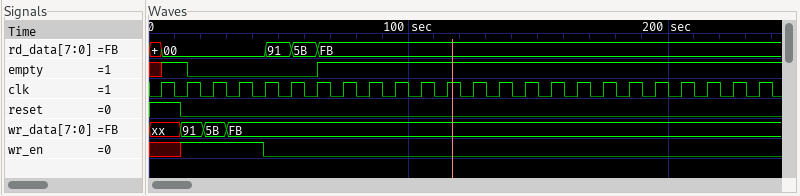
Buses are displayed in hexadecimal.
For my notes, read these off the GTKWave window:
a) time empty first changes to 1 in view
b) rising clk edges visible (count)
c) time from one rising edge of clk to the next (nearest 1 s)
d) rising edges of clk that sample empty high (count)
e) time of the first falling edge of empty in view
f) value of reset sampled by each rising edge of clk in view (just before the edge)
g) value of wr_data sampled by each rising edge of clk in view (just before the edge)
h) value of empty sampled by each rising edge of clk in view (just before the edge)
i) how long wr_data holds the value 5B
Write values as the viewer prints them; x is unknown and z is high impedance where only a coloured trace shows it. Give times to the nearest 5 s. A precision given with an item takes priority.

5 s
24
10 s
18
15 s
1 0 0 0 0 0 0 0 0 0 0 0 0 0 0 0 0 0 0 0 0 0 0 0
xx, 91, 5B, FB, FB, FB, FB, FB, FB, FB, FB, FB, FB, FB, FB, FB, FB, FB, FB, FB, FB, FB, FB, FB
x 1 0 0 0 0 0 1 1 1 1 1 1 1 1 1 1 1 1 1 1 1 1 1
10 s
